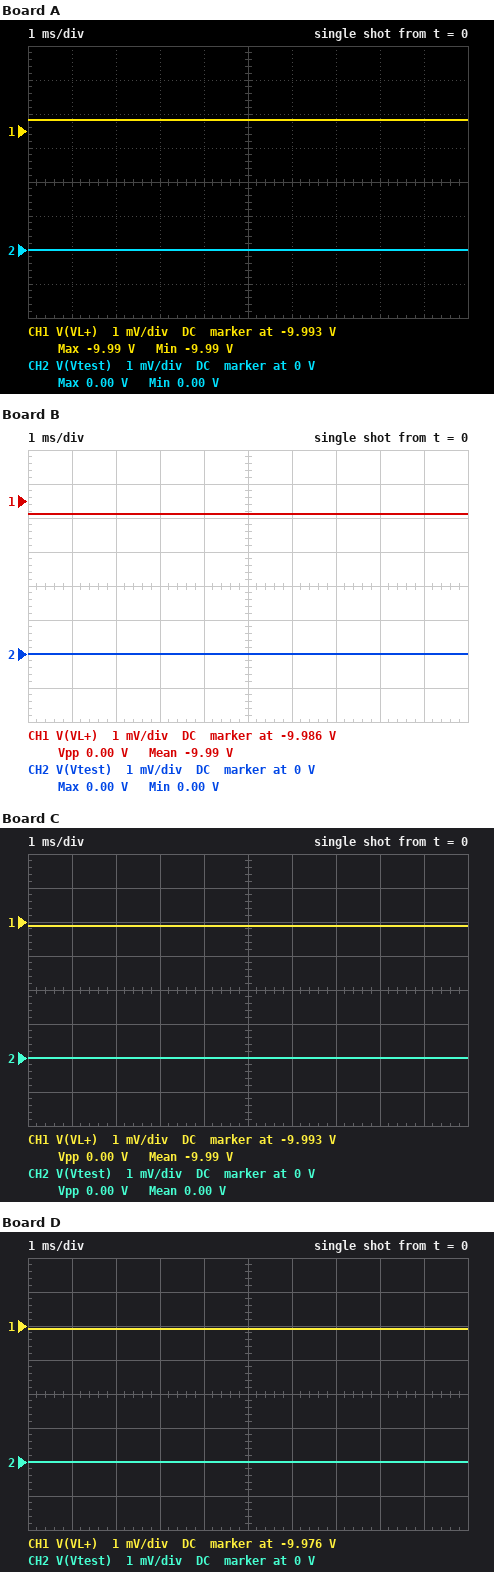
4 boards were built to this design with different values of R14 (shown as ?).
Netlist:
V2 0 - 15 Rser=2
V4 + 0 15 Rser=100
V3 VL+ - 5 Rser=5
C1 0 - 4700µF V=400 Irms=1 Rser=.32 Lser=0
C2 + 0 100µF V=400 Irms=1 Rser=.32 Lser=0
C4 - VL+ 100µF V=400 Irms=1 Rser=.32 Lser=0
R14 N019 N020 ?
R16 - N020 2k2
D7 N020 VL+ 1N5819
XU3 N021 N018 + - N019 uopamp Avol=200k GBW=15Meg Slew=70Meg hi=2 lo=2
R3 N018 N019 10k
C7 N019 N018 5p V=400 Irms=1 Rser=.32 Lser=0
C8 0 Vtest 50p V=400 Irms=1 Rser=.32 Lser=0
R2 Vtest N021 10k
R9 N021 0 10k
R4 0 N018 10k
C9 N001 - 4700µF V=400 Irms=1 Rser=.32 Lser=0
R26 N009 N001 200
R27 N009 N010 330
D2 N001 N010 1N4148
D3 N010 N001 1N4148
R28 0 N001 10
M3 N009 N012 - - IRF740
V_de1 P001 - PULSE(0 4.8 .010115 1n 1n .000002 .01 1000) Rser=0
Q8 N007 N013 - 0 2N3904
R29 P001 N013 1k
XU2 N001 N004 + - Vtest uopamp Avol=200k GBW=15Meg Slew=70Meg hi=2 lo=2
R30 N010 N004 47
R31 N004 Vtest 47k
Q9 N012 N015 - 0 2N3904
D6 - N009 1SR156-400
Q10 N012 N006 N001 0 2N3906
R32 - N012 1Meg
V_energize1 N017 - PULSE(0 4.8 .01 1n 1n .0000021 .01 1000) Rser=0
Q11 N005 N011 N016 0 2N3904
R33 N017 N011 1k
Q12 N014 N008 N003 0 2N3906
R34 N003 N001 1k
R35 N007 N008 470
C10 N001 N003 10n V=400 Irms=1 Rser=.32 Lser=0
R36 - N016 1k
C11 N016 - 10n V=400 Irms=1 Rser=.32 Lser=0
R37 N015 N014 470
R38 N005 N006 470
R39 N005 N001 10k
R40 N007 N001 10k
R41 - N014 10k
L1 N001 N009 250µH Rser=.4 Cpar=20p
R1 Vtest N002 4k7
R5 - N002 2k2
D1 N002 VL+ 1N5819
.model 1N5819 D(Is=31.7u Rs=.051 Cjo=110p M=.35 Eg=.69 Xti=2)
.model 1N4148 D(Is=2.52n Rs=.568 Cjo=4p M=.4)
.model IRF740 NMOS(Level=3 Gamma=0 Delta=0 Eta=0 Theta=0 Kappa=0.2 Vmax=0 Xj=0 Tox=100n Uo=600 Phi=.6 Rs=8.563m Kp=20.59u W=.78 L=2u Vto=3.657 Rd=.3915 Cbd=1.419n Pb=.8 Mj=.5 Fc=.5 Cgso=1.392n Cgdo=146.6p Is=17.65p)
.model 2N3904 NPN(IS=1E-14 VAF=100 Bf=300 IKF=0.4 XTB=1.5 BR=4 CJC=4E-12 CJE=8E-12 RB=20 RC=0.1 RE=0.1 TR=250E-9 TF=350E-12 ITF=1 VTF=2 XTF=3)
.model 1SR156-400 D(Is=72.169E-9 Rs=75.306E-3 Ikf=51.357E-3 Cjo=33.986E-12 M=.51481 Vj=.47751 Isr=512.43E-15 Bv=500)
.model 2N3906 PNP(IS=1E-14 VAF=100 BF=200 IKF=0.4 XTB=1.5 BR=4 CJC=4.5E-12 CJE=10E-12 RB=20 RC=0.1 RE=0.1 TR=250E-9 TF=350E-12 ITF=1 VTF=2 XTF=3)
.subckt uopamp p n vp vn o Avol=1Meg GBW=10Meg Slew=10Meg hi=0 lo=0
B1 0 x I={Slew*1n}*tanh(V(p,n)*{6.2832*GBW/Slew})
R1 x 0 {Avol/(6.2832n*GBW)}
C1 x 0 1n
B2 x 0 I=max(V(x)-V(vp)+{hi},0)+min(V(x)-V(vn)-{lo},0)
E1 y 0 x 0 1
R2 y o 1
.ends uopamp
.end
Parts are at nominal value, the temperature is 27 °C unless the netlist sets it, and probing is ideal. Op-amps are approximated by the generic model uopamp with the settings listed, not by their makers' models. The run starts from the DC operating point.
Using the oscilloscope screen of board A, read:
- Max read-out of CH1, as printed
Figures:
-9.99 V
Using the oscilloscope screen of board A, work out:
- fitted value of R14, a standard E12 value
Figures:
6.8 kΩ
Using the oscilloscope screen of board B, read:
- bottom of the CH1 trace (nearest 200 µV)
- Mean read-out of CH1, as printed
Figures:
-9.9864 V
-9.99 V
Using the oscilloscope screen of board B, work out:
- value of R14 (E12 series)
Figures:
3.3 kΩ
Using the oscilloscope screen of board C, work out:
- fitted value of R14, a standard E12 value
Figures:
8.2 kΩ
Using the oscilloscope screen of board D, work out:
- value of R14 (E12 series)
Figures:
2.2 kΩ
